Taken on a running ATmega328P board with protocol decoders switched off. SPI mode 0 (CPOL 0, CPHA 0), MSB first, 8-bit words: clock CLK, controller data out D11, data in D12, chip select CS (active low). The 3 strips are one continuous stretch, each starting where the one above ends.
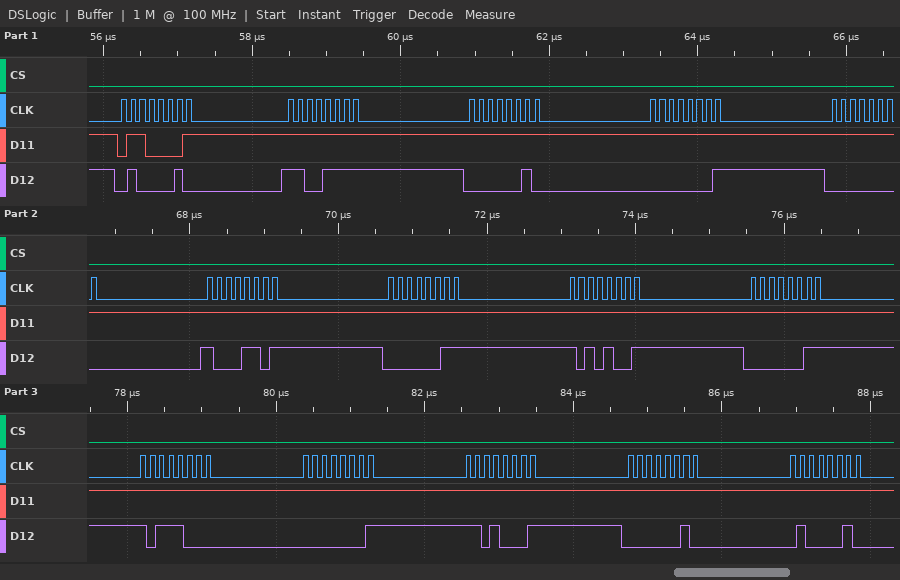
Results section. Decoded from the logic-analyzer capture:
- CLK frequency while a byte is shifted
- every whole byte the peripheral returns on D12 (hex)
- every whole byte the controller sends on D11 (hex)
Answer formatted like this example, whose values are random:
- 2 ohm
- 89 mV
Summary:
- 8 MHz
- 42 CF 02 01 00 8D 03 A9 03 B8 01 D1 02 42
- 61 FF FF FF FF FF FF FF FF FF FF FF FF FF
